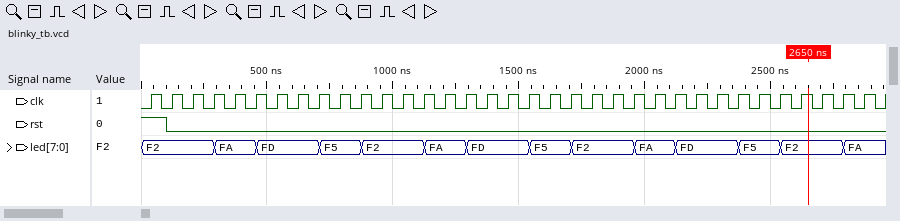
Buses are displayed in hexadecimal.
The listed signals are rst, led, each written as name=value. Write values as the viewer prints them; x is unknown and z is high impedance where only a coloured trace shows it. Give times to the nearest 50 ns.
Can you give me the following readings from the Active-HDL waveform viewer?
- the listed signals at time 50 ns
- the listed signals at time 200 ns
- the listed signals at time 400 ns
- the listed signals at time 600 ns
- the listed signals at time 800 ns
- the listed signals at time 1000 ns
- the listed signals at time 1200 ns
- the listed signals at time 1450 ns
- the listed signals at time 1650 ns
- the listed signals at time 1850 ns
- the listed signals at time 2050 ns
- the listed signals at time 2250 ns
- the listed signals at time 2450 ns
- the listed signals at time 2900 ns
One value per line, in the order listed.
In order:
rst=1, led=F2
rst=0, led=F2
rst=0, led=FA
rst=0, led=FD
rst=0, led=F5
rst=0, led=F2
rst=0, led=FA
rst=0, led=FD
rst=0, led=F5
rst=0, led=F2
rst=0, led=FA
rst=0, led=FD
rst=0, led=F5
rst=0, led=FA
